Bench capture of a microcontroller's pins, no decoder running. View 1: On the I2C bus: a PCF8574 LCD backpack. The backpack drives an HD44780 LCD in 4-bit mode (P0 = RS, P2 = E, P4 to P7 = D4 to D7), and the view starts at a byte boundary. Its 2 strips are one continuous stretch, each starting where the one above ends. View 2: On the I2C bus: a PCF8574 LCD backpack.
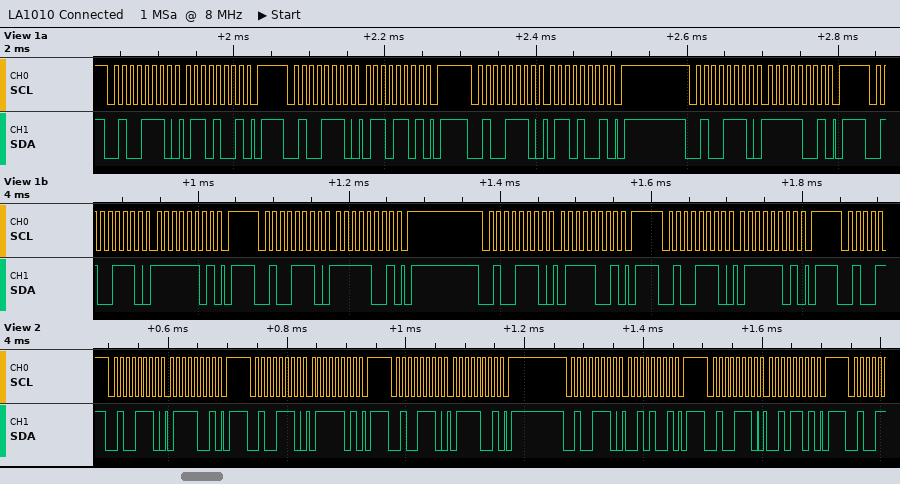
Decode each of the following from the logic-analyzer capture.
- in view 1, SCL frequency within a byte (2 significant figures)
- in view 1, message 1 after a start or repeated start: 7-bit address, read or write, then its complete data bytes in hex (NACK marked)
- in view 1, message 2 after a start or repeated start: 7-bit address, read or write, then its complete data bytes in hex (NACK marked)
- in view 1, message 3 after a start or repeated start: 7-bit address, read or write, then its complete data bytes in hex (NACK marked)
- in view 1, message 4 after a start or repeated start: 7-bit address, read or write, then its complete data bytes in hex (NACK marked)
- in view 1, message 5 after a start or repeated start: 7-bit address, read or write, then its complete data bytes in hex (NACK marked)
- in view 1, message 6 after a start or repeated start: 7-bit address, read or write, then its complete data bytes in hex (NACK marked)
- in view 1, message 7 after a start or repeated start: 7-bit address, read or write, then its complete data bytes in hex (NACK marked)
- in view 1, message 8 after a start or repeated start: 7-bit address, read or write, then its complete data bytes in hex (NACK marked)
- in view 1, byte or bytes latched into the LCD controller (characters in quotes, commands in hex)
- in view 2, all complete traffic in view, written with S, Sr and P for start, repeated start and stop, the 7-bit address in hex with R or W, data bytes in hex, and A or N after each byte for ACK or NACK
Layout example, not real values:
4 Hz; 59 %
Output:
100 kHz; 0x27 write: 69; 0x27 write: 6D; 0x27 write: 69; 0x27 write: F9; 0x27 write: FD; 0x27 write: F9; 0x27 write: 79; 0x27 write: 7D; 'o'; S 27W A 79 A P S 27W A 7D A P S 27W A 79 A P S 27W A 29 A P S 27W A 2D A P
